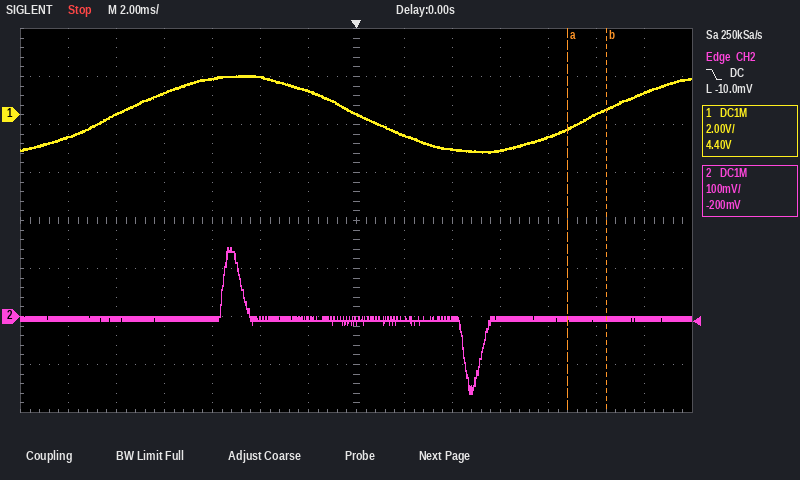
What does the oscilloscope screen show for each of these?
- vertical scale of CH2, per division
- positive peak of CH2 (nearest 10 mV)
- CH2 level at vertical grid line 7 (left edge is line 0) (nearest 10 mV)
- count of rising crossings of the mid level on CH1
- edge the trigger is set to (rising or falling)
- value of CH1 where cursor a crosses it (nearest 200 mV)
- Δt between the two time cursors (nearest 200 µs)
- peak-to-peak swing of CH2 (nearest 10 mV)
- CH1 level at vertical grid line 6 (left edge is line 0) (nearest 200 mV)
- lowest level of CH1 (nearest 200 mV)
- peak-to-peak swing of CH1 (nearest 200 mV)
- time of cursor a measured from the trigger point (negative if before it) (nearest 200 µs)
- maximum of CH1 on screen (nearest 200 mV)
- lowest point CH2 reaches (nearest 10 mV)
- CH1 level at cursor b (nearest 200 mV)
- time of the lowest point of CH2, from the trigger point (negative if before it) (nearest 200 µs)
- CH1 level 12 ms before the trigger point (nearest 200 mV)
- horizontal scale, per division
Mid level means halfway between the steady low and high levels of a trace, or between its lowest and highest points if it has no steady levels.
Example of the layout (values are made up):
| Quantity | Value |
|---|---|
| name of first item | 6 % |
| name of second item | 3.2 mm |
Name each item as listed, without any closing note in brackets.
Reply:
| Quantity | Value |
|---|---|
| vertical scale of CH2, per division | 100 mV |
| positive peak of CH2 | 140 mV |
| CH2 level at vertical grid line 7 (left edge is line 0) | -10 mV |
| count of rising crossings of the mid level on CH1 | 2 |
| edge the trigger is set to | falling |
| value of CH1 where cursor a crosses it | -600 mV |
| Δt between the two time cursors | 1.6 ms |
| peak-to-peak swing of CH2 | 300 mV |
| CH1 level at vertical grid line 6 (left edge is line 0) | 1.0 V |
| lowest level of CH1 | -1.6 V |
| peak-to-peak swing of CH1 | 3.2 V |
| time of cursor a measured from the trigger point (negative if before it) | +8.8 ms |
| maximum of CH1 on screen | 1.6 V |
| lowest point CH2 reaches | -160 mV |
| CH1 level at cursor b | 200 mV |
| time of the lowest point of CH2, from the trigger point (negative if before it) | +4.8 ms |
| CH1 level 12 ms before the trigger point | -1.0 V |
| horizontal scale, per division | 2 ms |
